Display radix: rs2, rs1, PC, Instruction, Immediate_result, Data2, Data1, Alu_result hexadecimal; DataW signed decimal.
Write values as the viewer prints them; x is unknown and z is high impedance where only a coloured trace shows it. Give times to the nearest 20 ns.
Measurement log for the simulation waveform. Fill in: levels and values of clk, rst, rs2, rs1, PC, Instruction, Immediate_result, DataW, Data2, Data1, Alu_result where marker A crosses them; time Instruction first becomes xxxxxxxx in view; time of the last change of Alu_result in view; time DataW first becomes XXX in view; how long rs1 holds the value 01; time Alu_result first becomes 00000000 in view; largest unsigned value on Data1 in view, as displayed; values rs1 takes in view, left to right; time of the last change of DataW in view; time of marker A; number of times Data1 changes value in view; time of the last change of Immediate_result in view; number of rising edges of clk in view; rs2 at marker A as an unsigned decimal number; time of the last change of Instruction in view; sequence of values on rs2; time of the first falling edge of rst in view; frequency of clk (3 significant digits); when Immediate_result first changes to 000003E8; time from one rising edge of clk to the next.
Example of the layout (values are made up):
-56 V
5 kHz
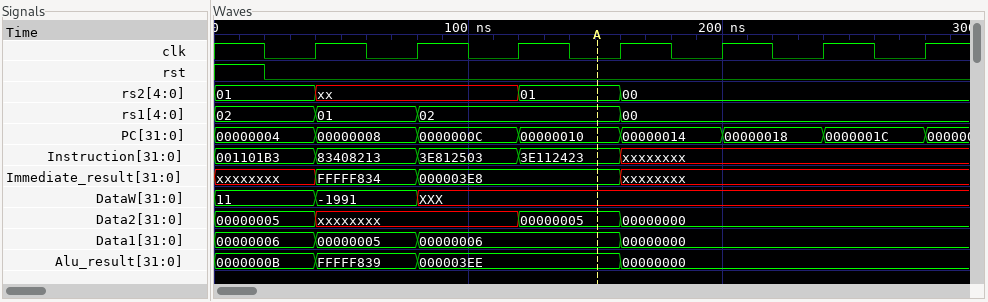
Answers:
clk=0, rst=0, rs2=01, rs1=02, PC=00000010, Instruction=3E112423, Immediate_result=000003E8, DataW=XXX, Data2=00000005, Data1=00000006, Alu_result=000003EE
160 ns
160 ns
80 ns
40 ns
160 ns
00000006
02, 01, 02, 00
80 ns
160 ns
3
160 ns
7
1
160 ns
01, xx, 01, 00
20 ns
25.0 MHz
80 ns
40 ns
